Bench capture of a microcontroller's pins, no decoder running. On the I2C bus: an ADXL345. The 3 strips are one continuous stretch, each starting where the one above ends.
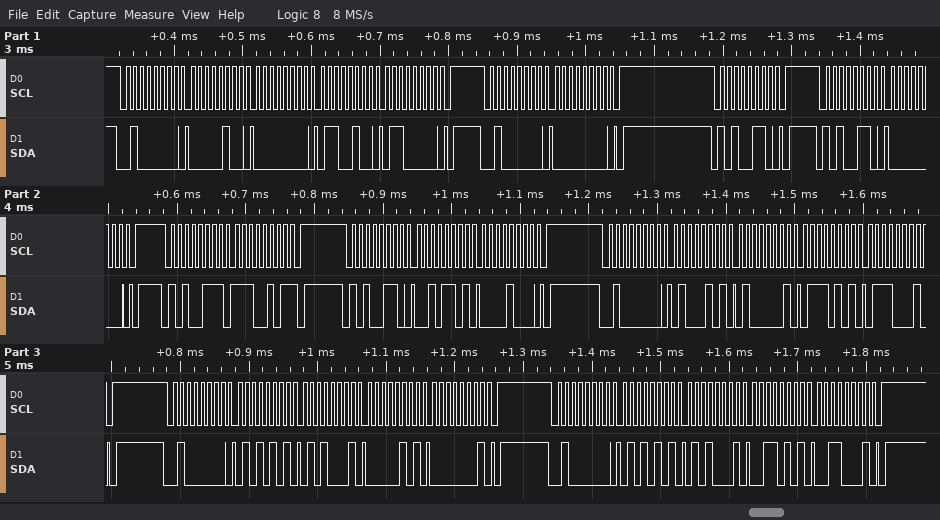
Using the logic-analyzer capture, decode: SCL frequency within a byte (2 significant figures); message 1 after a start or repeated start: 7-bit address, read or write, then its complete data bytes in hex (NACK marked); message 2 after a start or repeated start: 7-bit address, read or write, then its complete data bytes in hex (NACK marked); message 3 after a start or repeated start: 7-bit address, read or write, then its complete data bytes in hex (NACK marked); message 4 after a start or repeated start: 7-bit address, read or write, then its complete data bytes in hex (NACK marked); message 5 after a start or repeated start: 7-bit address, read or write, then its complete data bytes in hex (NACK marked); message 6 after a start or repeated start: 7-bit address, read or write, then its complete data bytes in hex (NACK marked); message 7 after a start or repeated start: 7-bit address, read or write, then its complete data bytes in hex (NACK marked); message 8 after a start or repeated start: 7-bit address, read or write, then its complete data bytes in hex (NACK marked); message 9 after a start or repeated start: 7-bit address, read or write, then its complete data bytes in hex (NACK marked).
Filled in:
100 kHz
0x20 write: 04 00 64 60
0x20 write: 00
0x53 write
0x53 write: 00
0x53 read: E5 NACK
0x53 write: 2D 08
0x20 write: 45 41 75 71
0x20 write: 55 51 05 01
0x20 write: 55 51 35 31
